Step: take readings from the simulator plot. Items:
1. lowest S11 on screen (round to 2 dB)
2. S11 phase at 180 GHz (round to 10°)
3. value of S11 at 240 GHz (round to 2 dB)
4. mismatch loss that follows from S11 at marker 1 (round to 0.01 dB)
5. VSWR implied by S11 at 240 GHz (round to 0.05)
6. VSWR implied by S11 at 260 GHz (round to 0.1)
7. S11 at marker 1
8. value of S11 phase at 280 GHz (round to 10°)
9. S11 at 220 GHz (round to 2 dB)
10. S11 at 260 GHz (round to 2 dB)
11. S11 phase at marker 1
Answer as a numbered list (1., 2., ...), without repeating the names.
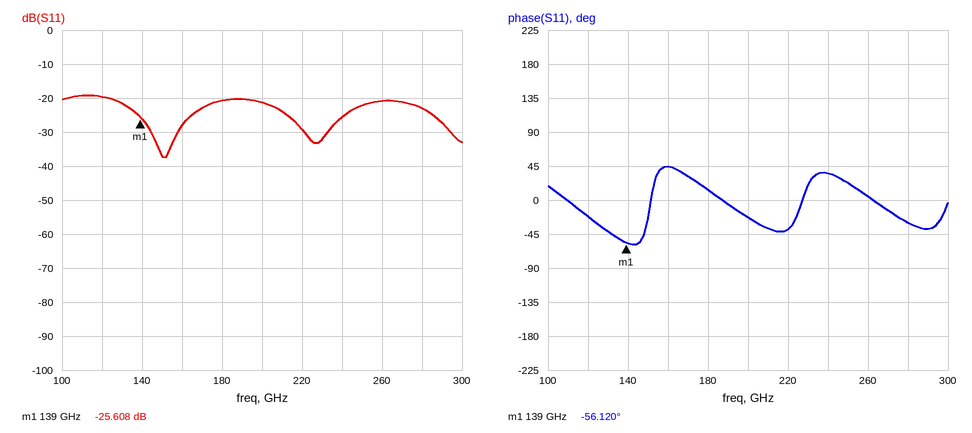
1. -38 dB
2. 10°
3. -26 dB
4. 0.01 dB
5. 1.10
6. 1.2
7. -25.608 dB
8. -30°
9. -30 dB
10. -20 dB
11. -56.120°
